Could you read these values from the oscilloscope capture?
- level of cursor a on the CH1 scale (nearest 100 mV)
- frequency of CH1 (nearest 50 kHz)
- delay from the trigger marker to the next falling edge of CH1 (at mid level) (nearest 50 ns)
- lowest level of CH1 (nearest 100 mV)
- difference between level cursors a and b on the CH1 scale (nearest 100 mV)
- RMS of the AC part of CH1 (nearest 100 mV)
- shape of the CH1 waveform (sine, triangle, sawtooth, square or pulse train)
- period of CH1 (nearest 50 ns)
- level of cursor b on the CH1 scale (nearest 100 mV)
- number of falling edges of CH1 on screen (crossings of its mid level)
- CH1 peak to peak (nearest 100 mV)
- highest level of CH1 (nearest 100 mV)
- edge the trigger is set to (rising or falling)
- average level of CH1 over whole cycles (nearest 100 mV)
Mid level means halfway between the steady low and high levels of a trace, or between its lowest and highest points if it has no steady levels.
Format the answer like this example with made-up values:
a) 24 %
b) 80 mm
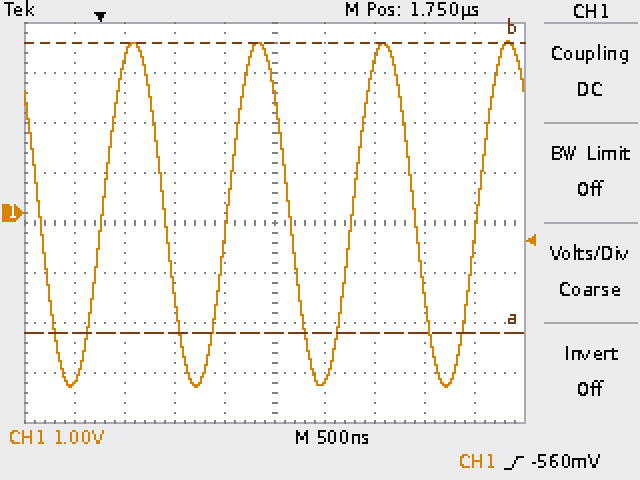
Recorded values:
a) -2.4 V
b) 800 kHz
c) 650 ns
d) -3.5 V
e) 5.8 V
f) 2.4 V
g) sine
h) 1.25 µs
i) 3.4 V
j) 4
k) 6.9 V
l) 3.4 V
m) rising
n) 0.0 V
